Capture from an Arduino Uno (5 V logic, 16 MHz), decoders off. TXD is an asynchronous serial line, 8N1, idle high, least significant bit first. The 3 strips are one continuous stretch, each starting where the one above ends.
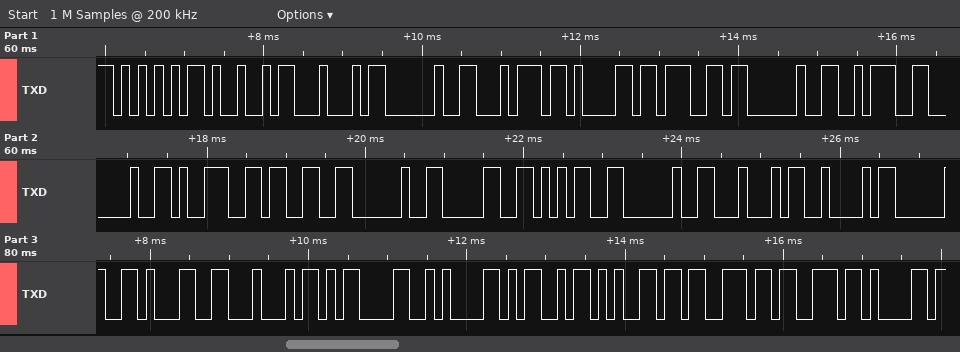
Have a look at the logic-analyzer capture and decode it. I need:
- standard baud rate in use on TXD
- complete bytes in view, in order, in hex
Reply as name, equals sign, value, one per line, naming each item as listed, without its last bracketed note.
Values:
standard baud rate in use on TXD = 9600 baud
complete bytes in view, in order, in hex = 55 49 44 20 74 61 67 20 3A 20 39 33 20 30 35 20 44 42 20 31 44 0D 0A 4D 65 73 73 61
